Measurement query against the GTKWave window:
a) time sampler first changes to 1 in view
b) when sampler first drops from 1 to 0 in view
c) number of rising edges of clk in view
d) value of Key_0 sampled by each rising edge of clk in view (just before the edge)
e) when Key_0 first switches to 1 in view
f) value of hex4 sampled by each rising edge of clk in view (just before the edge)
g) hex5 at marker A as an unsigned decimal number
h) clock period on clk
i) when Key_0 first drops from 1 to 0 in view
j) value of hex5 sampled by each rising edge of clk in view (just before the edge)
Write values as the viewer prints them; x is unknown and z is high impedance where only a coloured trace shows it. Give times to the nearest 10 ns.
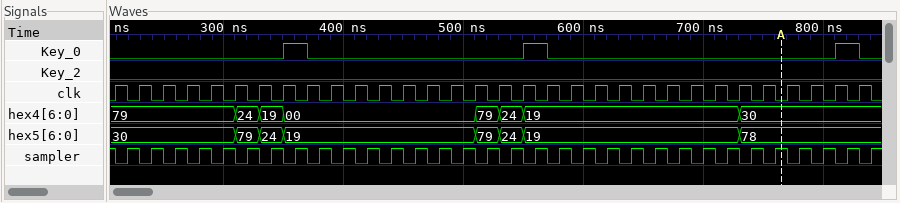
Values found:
220 ns
210 ns
32
0 0 0 0 0 0 0 0 1 0 0 0 0 0 0 0 0 0 1 0 0 0 0 0 0 0 0 0 0 0 0 1
350 ns
79, 79, 79, 79, 79, 79, 24, 19, 00, 00, 00, 00, 00, 00, 00, 00, 79, 24, 19, 19, 19, 19, 19, 19, 19, 19, 19, 30, 30, 30, 30, 30
120
20 ns
370 ns
30, 30, 30, 30, 30, 30, 79, 24, 19, 19, 19, 19, 19, 19, 19, 19, 79, 24, 19, 19, 19, 19, 19, 19, 19, 19, 19, 78, 78, 78, 78, 78
